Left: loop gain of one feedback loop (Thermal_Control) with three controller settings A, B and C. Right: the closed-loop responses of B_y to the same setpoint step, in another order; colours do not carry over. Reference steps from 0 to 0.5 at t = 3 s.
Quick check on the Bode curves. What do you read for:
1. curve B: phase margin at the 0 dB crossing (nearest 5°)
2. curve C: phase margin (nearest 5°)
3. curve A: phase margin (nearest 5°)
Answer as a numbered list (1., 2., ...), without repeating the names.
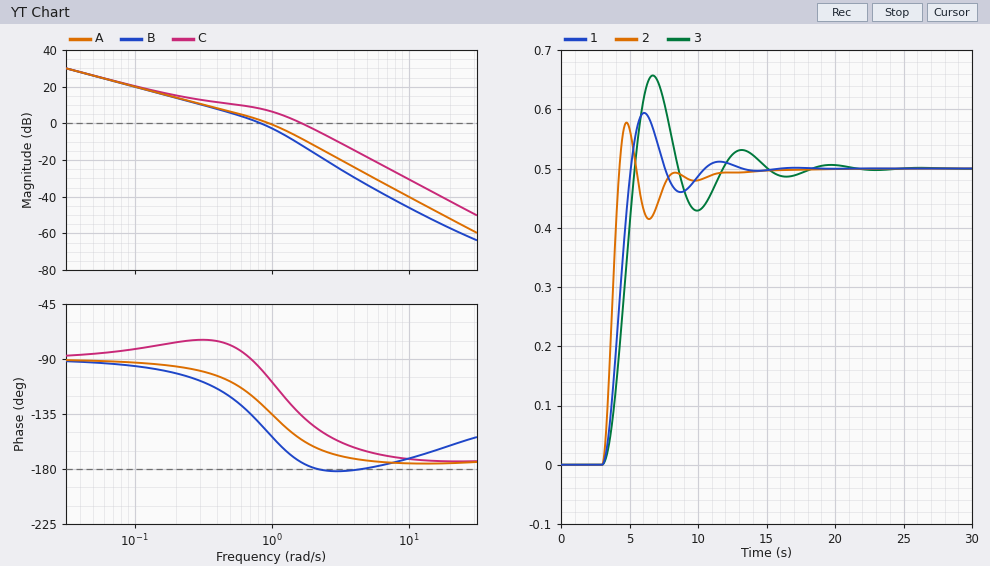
1. 35°
2. 45°
3. 45°
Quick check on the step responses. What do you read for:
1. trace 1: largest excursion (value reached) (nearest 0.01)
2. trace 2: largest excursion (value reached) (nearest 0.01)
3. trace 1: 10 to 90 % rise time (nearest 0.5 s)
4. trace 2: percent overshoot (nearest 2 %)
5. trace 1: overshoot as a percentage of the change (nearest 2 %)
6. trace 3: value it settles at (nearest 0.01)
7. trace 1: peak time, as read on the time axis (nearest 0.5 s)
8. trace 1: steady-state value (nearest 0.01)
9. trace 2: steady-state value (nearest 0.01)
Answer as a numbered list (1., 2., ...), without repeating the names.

1. 0.59
2. 0.58
3. 1.5 s
4. 16 %
5. 18 %
6. 0.50
7. 6.0 s
8. 0.50
9. 0.50
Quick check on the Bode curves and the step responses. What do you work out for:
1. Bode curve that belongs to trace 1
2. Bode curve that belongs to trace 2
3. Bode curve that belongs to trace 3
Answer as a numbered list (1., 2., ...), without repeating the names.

1. A
2. C
3. B
